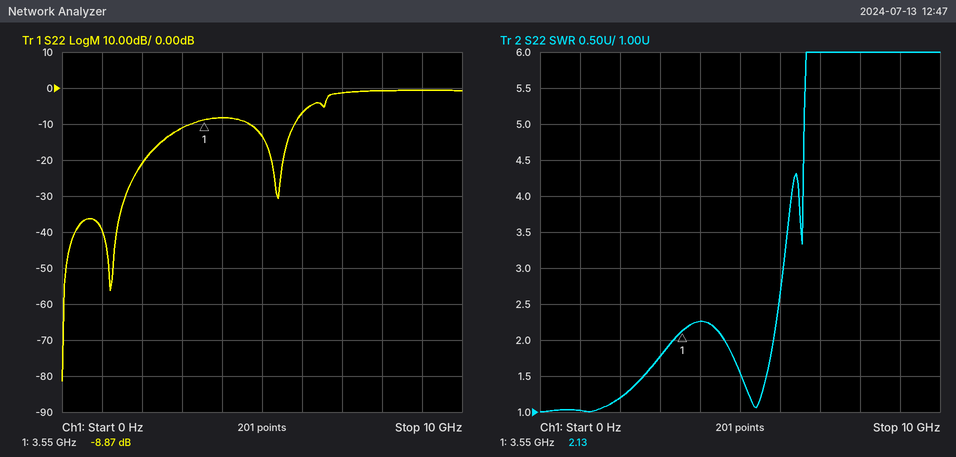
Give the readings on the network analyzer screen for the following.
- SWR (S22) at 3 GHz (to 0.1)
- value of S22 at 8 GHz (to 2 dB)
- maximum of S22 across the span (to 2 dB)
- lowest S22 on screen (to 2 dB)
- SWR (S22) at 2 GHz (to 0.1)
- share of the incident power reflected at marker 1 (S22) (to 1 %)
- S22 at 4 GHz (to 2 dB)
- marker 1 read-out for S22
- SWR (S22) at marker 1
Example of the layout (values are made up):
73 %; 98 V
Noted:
1.8; 0 dB; 0 dB; -82 dB; 1.2; 13 %; -8 dB; -8.87 dB; 2.13
